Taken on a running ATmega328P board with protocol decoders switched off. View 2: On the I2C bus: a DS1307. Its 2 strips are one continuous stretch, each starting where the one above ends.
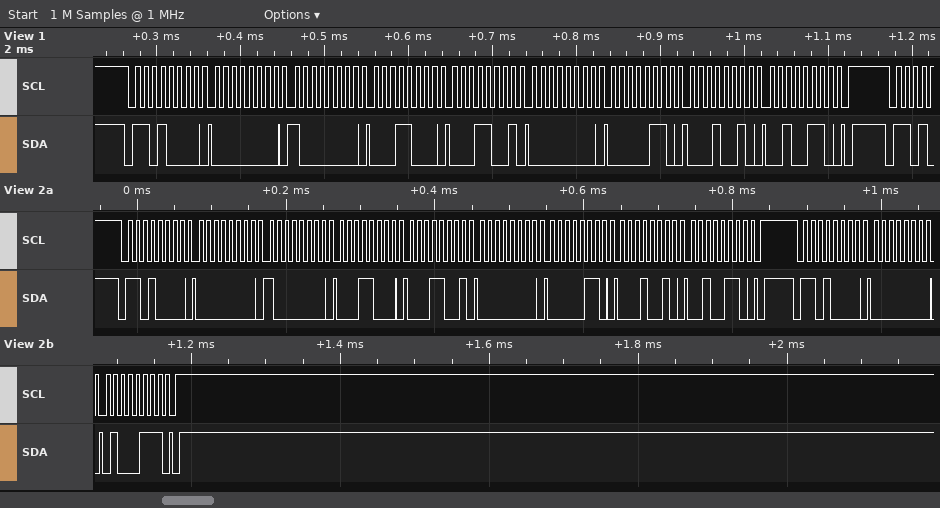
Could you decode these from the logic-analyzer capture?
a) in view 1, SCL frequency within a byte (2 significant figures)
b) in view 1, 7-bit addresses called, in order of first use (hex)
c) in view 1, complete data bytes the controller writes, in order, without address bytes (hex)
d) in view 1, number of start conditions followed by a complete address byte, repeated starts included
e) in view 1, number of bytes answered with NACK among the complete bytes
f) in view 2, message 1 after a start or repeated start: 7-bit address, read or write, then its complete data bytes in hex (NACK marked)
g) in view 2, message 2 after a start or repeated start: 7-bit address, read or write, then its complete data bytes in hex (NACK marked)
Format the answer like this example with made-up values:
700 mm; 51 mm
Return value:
100 kHz; 0x68; 00 80 18 19 00 06 12 26; 1; 0; 0x68 write: 00 80 18 19 00 06 12 26; 0x68 write: 00 47
